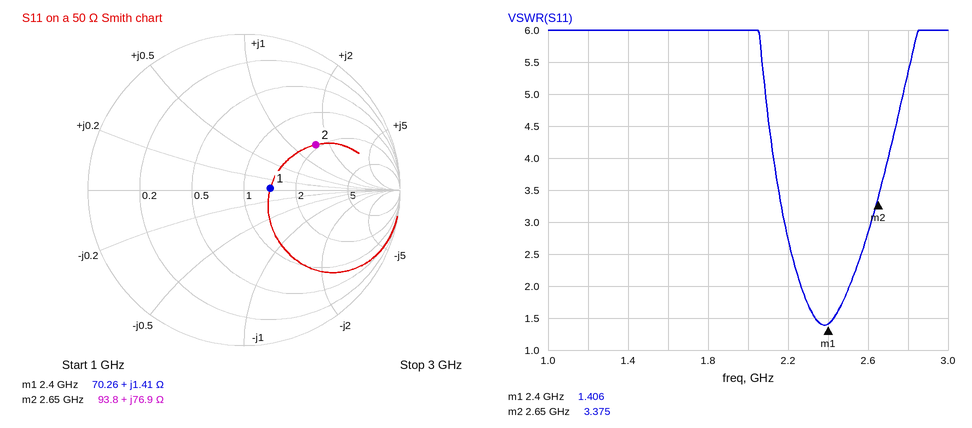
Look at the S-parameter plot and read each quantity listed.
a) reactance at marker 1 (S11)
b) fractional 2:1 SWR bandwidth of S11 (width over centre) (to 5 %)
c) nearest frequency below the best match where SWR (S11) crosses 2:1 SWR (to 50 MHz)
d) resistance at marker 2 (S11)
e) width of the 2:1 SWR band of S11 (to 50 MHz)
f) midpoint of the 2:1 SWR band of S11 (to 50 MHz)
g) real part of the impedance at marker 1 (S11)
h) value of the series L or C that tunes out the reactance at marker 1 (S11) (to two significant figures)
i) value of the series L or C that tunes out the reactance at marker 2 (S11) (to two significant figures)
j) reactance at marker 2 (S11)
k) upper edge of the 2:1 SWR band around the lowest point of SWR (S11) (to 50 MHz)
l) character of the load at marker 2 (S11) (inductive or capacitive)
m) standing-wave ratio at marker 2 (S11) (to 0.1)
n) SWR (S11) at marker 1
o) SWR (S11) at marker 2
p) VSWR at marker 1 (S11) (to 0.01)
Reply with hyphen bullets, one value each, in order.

- +1.41 Ω
- 10 %
- 2.25 GHz
- 93.8 Ω
- 250 MHz
- 2.40 GHz
- 70.26 Ω
- 47 pF
- 780 fF
- +76.9 Ω
- 2.50 GHz
- inductive
- 3.4
- 1.406
- 3.375
- 1.41
